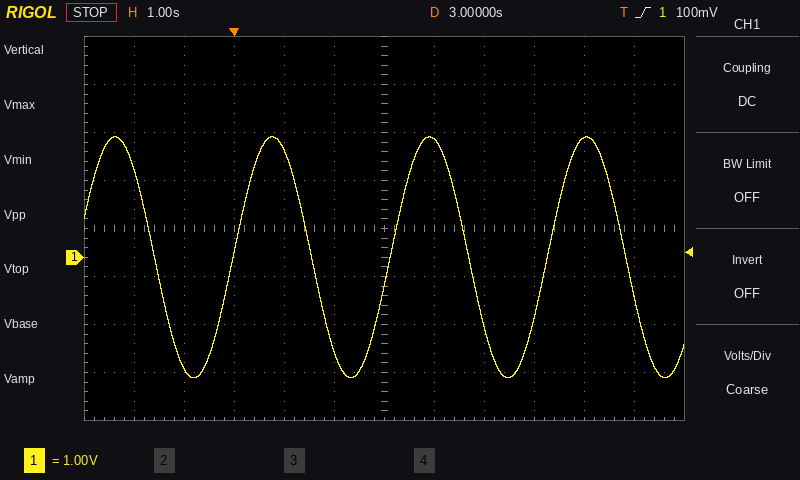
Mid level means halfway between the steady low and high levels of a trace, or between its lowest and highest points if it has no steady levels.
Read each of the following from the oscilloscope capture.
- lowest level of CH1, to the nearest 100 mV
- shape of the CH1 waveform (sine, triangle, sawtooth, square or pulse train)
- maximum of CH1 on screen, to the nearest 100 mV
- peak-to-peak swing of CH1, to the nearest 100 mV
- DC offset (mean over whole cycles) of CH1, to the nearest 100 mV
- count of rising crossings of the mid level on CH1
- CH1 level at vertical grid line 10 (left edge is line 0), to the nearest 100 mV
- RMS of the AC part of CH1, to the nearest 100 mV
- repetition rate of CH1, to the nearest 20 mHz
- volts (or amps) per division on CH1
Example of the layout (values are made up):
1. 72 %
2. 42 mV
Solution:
1. -2.5 V
2. sine
3. 2.5 V
4. 5.0 V
5. 0.0 V
6. 3
7. 2.5 V
8. 1.8 V
9. 320 mHz
10. 1 V
